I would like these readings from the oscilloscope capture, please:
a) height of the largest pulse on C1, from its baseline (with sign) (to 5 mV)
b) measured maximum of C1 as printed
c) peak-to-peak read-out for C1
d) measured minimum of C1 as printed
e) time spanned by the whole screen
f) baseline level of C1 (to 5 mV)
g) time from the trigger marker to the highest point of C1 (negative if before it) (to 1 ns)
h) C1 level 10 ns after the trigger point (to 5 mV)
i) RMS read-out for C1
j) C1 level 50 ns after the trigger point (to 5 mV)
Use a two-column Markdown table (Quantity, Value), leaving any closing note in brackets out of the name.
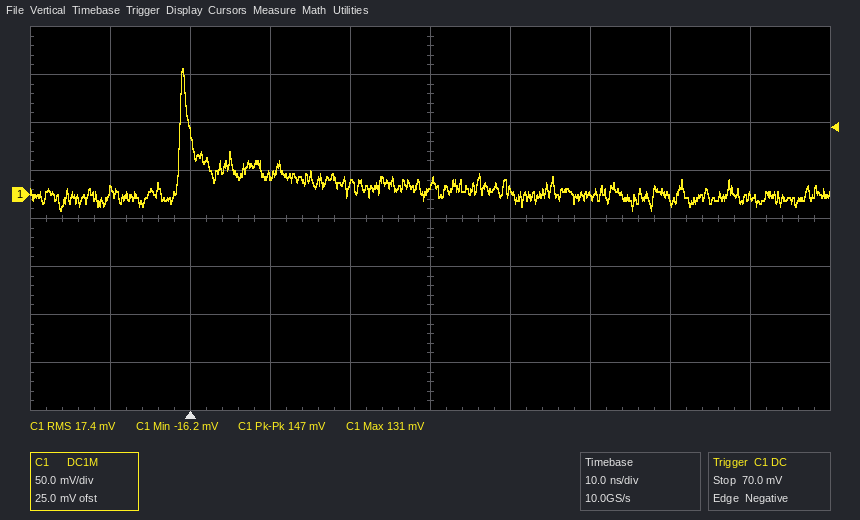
| Quantity | Value |
|---|---|
| height of the largest pulse on C1, from its baseline (with sign) | +130 mV |
| measured maximum of C1 as printed | 131 mV |
| peak-to-peak read-out for C1 | 147 mV |
| measured minimum of C1 as printed | -16.2 mV |
| time spanned by the whole screen | 100 ns |
| baseline level of C1 | 0 mV |
| time from the trigger marker to the highest point of C1 (negative if before it) | -1 ns |
| C1 level 10 ns after the trigger point | 20 mV |
| RMS read-out for C1 | 17.4 mV |
| C1 level 50 ns after the trigger point | 0 mV |
